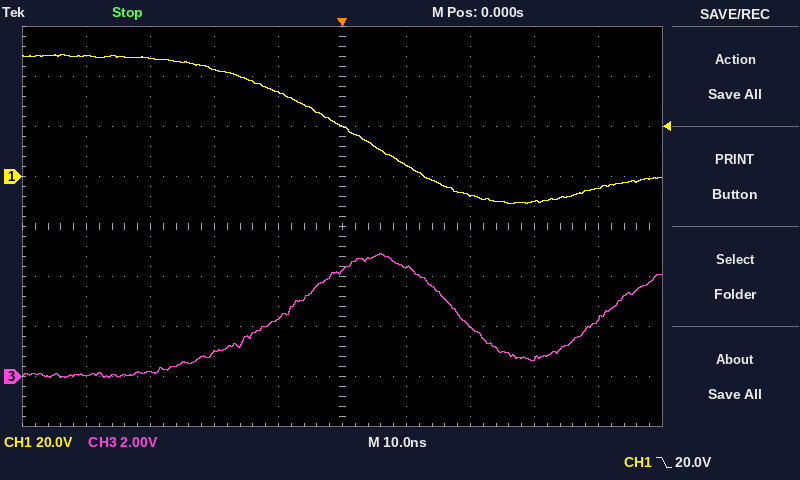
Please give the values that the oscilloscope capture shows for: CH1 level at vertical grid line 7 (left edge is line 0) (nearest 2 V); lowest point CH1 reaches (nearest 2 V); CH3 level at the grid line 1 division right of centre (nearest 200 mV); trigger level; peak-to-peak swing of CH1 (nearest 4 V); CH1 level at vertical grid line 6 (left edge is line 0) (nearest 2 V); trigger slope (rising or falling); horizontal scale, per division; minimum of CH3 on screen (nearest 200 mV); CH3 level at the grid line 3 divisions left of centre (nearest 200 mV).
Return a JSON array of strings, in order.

["-8 V", "-10 V", "4.4 V", "20.0 V", "60 V", "4 V", "falling", "10 ns", "0.0 V", "200 mV"]
